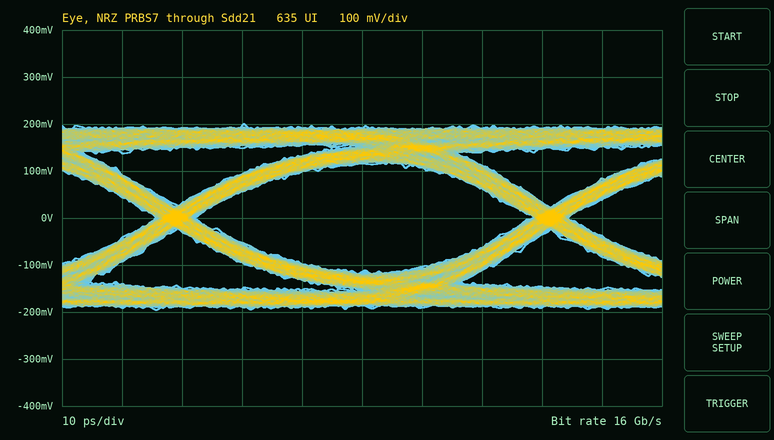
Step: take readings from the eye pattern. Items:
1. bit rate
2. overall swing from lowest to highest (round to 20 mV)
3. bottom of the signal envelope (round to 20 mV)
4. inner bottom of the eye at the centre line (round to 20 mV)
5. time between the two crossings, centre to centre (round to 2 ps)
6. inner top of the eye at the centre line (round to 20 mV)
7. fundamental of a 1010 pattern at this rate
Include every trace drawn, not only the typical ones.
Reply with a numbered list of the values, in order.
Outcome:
1. 16 Gb/s
2. 400 mV
3. -200 mV
4. -120 mV
5. 62 ps
6. 120 mV
7. 8 GHz
